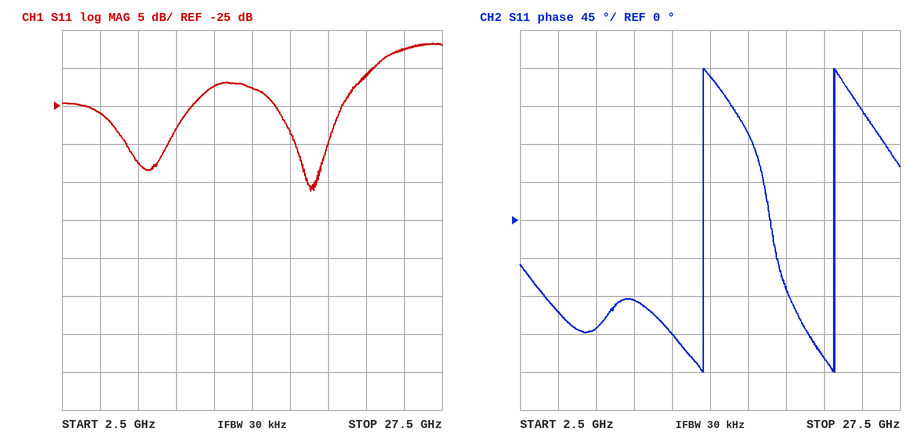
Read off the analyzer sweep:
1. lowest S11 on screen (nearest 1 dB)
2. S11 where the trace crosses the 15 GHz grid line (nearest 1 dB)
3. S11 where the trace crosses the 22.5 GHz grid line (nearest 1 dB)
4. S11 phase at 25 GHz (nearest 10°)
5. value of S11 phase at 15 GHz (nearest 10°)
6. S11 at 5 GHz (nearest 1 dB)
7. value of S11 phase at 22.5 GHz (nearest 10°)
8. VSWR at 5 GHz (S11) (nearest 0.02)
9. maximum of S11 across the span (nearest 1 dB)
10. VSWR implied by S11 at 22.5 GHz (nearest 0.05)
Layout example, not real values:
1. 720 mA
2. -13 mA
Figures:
1. -36 dB
2. -23 dB
3. -21 dB
4. 130°
5. 170°
6. -26 dB
7. -160°
8. 1.10
9. -17 dB
10. 1.20
